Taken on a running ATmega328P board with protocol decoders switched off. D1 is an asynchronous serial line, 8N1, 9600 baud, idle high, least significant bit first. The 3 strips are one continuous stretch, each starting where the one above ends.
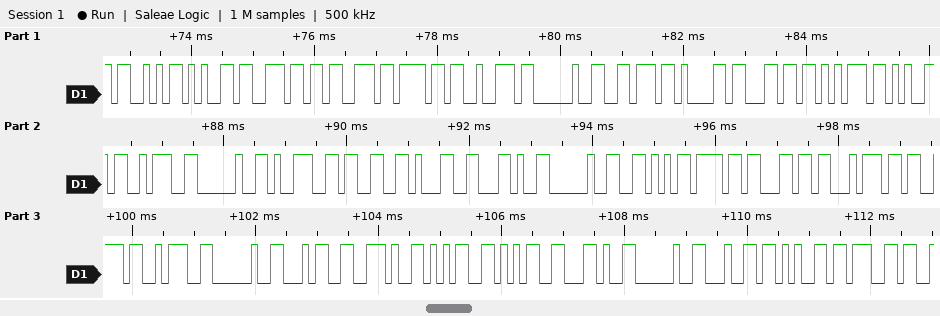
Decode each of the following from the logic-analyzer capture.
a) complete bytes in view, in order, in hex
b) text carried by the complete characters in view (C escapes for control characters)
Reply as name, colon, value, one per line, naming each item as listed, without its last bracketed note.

complete bytes in view, in order, in hex: 53 65 6E 73 6F 72 20 76 61 6C 75 65 3A 20 39 33 31 2C 20 56 6F 6C 74 73 3A 20 34 2E 35 35 2C 20 64 65 67
text carried by the complete characters in view: "Sensor value: 931, Volts: 4.55, deg"
